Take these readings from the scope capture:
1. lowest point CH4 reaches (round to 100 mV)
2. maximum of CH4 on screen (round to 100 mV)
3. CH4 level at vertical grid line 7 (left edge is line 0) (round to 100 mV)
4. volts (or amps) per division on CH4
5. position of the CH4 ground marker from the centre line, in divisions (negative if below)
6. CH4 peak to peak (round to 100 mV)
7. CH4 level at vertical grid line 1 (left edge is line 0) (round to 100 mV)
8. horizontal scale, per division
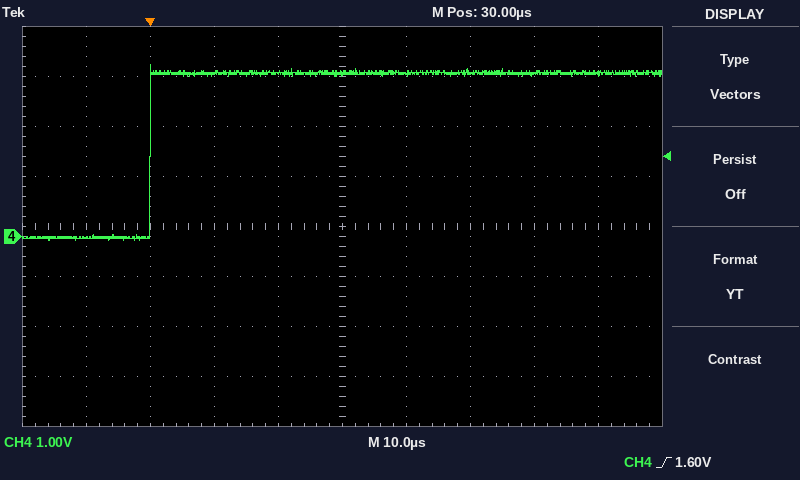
-100 mV
3.4 V
3.3 V
1 V
-0.2 div
3.5 V
0.0 V
10 µs
